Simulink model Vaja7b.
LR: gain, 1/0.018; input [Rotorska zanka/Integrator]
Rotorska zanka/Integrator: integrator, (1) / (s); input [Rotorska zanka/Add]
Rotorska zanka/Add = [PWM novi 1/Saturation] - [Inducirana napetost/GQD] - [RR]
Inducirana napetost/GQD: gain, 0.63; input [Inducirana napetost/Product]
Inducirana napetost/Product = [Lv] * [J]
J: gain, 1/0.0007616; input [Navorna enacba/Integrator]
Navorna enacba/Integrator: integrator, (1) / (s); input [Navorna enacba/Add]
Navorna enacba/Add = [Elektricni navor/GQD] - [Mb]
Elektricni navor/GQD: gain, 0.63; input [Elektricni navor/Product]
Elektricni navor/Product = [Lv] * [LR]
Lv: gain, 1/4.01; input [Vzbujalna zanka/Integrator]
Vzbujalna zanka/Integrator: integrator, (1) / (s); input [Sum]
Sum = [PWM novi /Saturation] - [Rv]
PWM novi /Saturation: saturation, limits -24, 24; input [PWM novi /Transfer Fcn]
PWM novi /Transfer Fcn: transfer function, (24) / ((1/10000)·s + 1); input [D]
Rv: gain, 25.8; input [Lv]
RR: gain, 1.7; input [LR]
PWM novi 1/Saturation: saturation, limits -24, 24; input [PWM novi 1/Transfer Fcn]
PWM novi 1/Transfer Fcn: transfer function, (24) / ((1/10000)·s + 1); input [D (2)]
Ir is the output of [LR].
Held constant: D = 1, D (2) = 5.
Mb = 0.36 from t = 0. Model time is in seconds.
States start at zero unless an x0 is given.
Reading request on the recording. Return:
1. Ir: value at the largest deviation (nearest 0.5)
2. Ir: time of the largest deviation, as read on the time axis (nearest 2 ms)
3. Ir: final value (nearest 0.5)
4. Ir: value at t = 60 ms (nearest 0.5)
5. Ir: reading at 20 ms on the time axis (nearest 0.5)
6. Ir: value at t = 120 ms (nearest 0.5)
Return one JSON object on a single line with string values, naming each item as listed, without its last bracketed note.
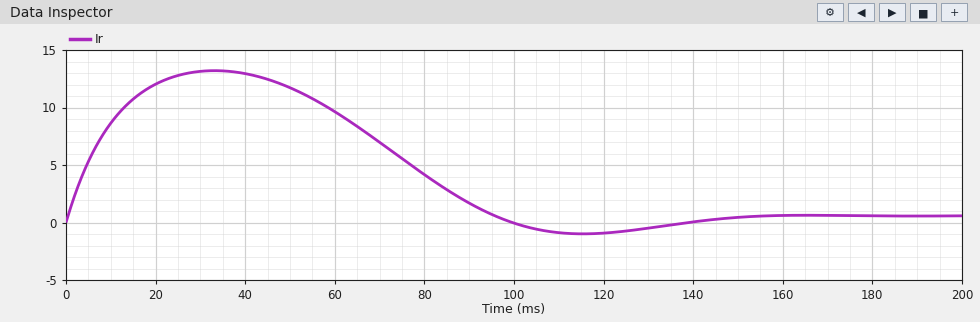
{"Ir: value at the largest deviation": "13.0", "Ir: time of the largest deviation, as read on the time axis": "34 ms", "Ir: final value": "0.5", "Ir: value at t = 60 ms": "9.5", "Ir: reading at 20 ms on the time axis": "12.0", "Ir: value at t = 120 ms": "-1.0"}
